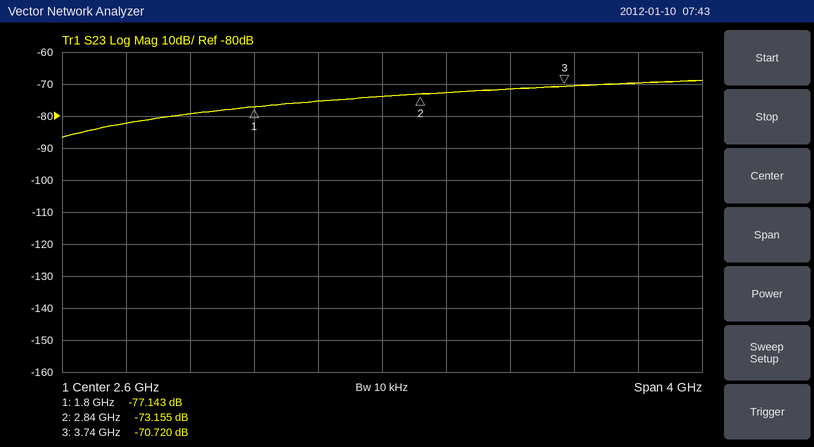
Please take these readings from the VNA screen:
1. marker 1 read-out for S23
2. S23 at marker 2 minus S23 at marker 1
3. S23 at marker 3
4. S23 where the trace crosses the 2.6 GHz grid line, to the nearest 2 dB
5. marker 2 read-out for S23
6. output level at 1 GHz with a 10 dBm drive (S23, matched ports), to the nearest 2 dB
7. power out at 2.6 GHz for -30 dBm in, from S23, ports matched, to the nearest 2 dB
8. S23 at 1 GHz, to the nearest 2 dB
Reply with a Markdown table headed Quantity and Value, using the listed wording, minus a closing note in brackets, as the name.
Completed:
| Quantity | Value |
|---|---|
| marker 1 read-out for S23 | -77.143 dB |
| S23 at marker 2 minus S23 at marker 1 | 3.988 dB |
| S23 at marker 3 | -70.720 dB |
| S23 where the trace crosses the 2.6 GHz grid line, to the nearest 2 dB | -74 dB |
| marker 2 read-out for S23 | -73.155 dB |
| output level at 1 GHz with a 10 dBm drive (S23, matched ports), to the nearest 2 dB | -72 dBm |
| power out at 2.6 GHz for -30 dBm in, from S23, ports matched, to the nearest 2 dB | -104 dBm |
| S23 at 1 GHz, to the nearest 2 dB | -82 dB |
